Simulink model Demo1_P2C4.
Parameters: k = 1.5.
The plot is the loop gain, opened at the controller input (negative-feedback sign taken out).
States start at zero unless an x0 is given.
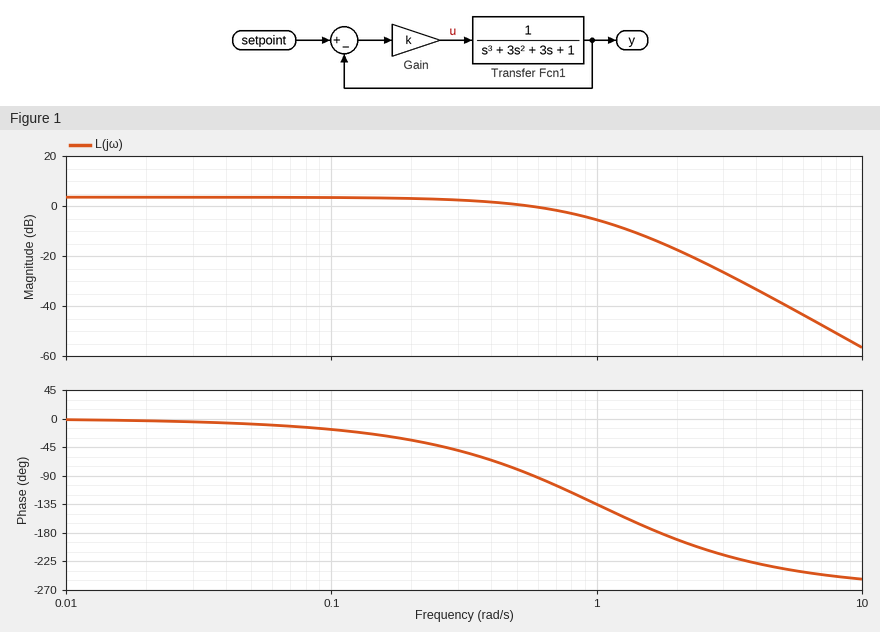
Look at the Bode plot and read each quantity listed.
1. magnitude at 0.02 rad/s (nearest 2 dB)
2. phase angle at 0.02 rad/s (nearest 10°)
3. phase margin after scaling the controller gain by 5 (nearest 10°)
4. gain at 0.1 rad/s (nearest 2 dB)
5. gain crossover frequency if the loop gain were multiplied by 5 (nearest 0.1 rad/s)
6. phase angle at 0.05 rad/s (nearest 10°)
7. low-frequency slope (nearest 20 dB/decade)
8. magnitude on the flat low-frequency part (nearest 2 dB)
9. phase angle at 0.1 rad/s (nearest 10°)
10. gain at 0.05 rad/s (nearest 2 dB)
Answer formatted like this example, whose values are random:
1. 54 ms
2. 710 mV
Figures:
1. 4 dB
2. 0°
3. 0°
4. 4 dB
5. 1.7 rad/s
6. -10°
7. 0 dB/decade
8. 4 dB
9. -20°
10. 4 dB
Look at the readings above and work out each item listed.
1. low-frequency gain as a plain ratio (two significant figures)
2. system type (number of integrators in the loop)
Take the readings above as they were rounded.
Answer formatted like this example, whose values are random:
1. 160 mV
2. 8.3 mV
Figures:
1. 1.6
2. 0
